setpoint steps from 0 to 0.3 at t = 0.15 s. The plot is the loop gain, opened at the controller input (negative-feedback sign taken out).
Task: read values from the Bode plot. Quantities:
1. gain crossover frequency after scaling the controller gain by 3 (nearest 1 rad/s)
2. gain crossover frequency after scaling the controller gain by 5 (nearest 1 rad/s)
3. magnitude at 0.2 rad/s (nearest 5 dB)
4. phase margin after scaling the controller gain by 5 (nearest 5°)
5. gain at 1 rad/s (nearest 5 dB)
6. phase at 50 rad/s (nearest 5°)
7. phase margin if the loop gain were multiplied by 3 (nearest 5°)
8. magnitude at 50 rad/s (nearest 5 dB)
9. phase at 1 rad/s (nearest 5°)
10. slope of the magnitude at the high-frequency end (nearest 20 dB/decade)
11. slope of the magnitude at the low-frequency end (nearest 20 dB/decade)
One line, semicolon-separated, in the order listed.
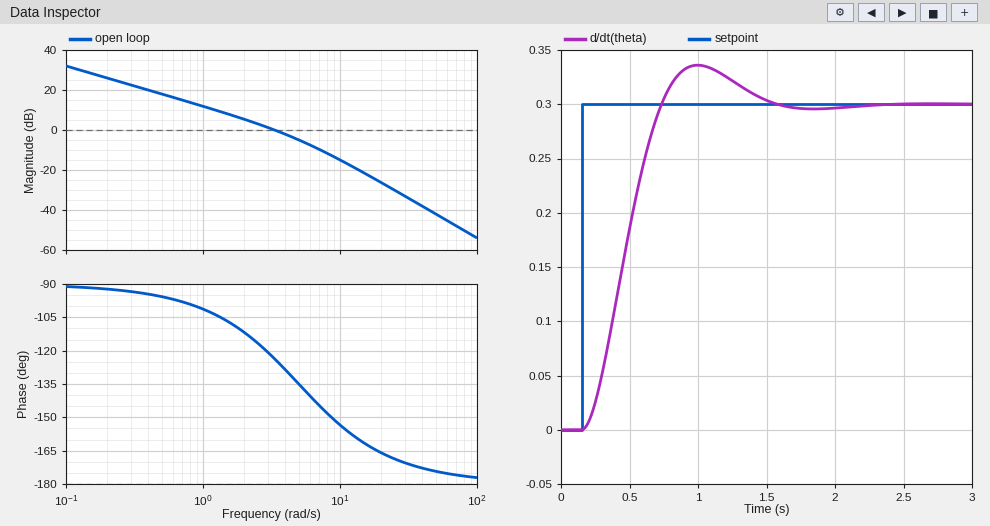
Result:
7 rad/s; 9 rad/s; 25 dB; 30°; 10 dB; -175°; 35°; -40 dB; -100°; -40 dB/decade; -20 dB/decade
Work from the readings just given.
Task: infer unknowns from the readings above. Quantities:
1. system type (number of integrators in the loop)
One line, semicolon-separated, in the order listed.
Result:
1
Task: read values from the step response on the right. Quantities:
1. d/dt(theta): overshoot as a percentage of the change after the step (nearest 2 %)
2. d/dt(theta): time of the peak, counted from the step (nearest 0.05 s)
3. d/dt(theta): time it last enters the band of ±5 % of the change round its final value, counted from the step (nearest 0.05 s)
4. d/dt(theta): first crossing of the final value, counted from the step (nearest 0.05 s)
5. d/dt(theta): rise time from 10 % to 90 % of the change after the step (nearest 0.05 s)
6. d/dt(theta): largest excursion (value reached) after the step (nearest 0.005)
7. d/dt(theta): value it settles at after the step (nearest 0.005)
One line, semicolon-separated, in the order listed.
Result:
12 %; 0.85 s; 1.20 s; 0.60 s; 0.40 s; 0.335; 0.300
